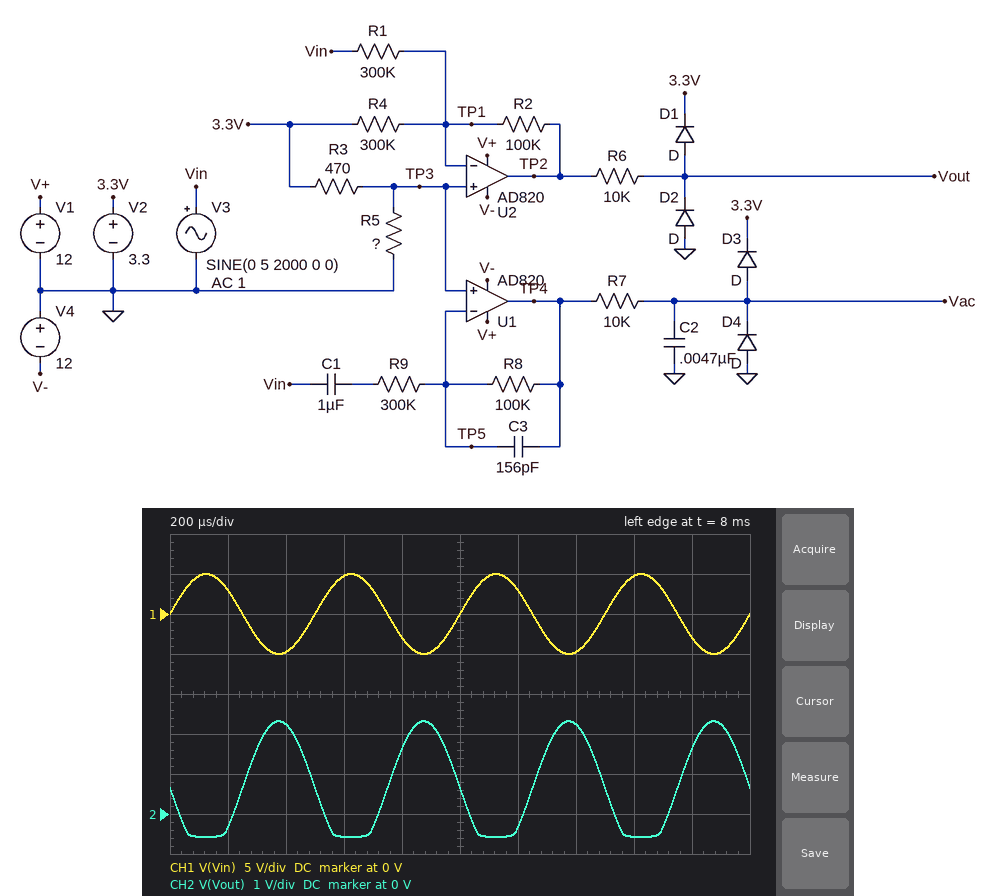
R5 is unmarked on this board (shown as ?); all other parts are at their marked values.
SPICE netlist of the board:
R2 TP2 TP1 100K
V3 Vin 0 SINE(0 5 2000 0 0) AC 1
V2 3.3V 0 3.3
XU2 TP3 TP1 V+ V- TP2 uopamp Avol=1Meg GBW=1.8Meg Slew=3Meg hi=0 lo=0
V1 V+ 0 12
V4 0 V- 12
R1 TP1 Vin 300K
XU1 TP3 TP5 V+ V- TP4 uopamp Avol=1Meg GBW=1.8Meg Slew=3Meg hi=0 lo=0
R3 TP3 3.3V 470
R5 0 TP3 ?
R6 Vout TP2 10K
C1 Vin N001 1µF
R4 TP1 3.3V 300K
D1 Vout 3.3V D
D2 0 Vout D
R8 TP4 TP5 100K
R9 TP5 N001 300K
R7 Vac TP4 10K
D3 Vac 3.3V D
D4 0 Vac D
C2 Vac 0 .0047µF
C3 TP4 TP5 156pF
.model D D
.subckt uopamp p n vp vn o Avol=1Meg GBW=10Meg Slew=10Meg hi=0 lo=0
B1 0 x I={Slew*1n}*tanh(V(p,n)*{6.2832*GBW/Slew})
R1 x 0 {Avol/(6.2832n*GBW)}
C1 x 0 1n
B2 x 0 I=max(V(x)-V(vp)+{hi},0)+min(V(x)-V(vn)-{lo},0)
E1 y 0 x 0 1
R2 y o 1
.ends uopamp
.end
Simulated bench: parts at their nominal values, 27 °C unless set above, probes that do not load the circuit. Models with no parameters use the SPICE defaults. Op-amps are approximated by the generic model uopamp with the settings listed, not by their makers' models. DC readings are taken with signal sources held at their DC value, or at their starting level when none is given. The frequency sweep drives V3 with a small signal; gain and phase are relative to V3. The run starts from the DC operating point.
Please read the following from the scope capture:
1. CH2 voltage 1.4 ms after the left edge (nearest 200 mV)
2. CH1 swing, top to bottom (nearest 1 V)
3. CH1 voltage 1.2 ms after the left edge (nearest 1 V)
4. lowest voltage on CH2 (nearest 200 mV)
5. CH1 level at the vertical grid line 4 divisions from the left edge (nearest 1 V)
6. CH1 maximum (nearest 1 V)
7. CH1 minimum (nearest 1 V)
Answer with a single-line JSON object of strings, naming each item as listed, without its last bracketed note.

{"CH2 voltage 1.4 ms after the left edge": "2.2 V", "CH1 swing, top to bottom": "10 V", "CH1 voltage 1.2 ms after the left edge": "3 V", "lowest voltage on CH2": "-600 mV", "CH1 level at the vertical grid line 4 divisions from the left edge": "-3 V", "CH1 maximum": "5 V", "CH1 minimum": "-5 V"}
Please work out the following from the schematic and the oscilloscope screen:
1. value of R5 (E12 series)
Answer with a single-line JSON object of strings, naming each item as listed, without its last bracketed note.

{"value of R5": "220 Ω"}
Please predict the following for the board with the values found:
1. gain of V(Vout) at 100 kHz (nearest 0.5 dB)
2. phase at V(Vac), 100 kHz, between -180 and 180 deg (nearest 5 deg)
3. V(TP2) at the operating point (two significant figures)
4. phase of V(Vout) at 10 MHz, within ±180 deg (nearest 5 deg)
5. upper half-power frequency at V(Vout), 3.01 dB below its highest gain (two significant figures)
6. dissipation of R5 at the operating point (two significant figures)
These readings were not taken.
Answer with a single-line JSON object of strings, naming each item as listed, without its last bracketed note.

{"gain of V(Vout) at 100 kHz": "-9.5 dB", "phase at V(Vac), 100 kHz, between -180 and 180 deg": "5 deg", "V(TP2) at the operating point": "650 mV", "phase of V(Vout) at 10 MHz, within ±180 deg": "95 deg", "upper half-power frequency at V(Vout), 3.01 dB below its highest gain": "1.1 MHz", "dissipation of R5 at the operating point": "5.0 mW"}
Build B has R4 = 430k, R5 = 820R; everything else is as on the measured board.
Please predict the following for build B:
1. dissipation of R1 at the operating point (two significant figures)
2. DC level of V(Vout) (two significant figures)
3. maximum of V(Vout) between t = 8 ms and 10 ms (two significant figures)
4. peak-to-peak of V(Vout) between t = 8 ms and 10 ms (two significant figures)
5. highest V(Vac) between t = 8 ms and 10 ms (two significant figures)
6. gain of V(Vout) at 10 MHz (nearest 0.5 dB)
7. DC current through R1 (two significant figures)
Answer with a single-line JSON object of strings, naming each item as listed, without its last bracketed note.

{"dissipation of R1 at the operating point": "15 µW", "DC level of V(Vout)": "2.5 V", "maximum of V(Vout) between t = 8 ms and 10 ms": "3.9 V", "peak-to-peak of V(Vout) between t = 8 ms and 10 ms": "3.0 V", "highest V(Vac) between t = 8 ms and 10 ms": "3.5 V", "gain of V(Vout) at 10 MHz": "-28.5 dB", "DC current through R1": "7.0 µA"}
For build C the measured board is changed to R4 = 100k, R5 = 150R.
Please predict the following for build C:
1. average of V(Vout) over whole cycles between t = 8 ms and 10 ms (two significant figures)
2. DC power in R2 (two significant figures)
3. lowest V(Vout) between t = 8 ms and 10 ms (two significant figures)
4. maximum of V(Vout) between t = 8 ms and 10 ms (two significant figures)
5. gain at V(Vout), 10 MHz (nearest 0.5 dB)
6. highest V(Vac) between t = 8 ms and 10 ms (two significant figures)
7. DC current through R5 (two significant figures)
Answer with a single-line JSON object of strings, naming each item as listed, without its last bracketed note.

{"average of V(Vout) over whole cycles between t = 8 ms and 10 ms": "-420 mV", "DC power in R2": "50 µW", "lowest V(Vout) between t = 8 ms and 10 ms": "-620 mV", "maximum of V(Vout) between t = 8 ms and 10 ms": "230 mV", "gain at V(Vout), 10 MHz": "-62.5 dB", "highest V(Vac) between t = 8 ms and 10 ms": "2.2 V", "DC current through R5": "5.3 mA"}
